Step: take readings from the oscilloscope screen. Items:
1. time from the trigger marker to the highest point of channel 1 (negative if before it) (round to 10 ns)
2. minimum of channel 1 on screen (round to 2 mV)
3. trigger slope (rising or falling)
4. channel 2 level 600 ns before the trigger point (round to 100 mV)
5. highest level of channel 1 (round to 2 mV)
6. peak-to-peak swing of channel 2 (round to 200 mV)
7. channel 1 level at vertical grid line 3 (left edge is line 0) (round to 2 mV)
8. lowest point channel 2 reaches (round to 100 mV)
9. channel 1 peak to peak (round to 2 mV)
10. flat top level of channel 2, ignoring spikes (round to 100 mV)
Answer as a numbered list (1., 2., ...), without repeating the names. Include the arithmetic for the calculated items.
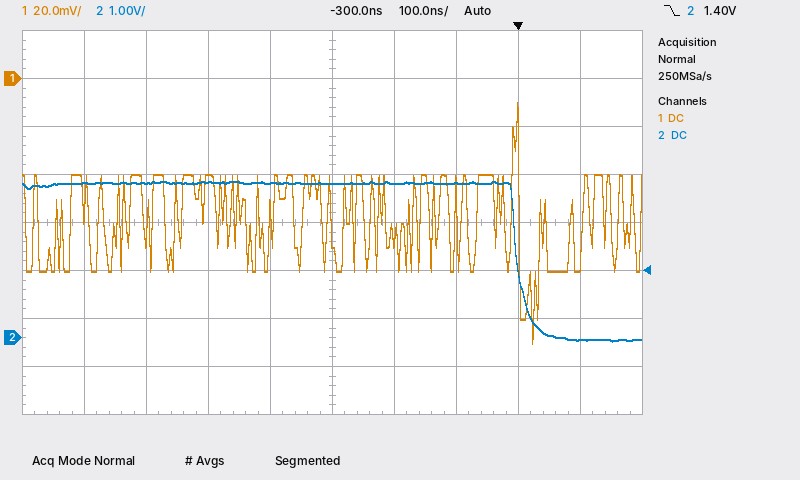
1. 0 ns
2. -110 mV
3. falling
4. 3.2 V
5. -10 mV
6. 3.4 V
7. -42 mV
8. -100 mV
9. -10 mV − (-110 mV) = 100 mV
10. 3.2 V
